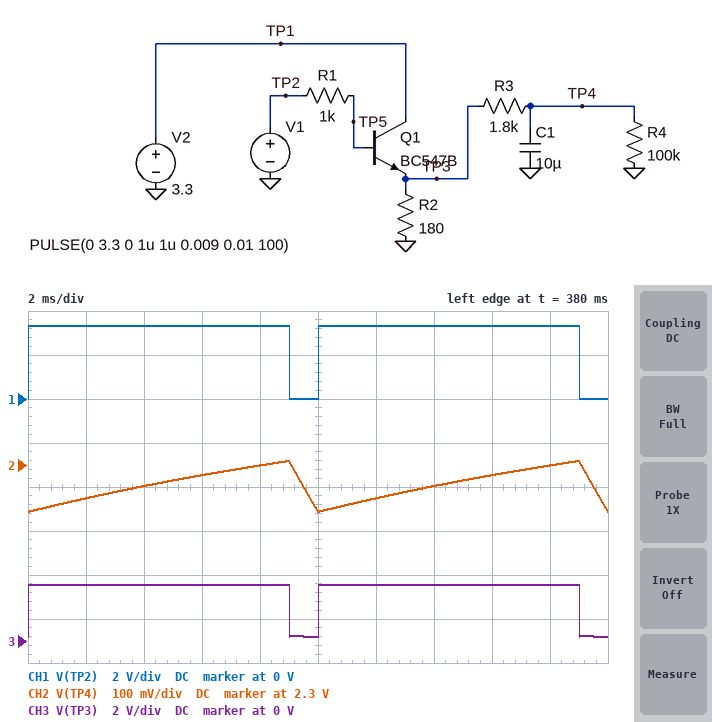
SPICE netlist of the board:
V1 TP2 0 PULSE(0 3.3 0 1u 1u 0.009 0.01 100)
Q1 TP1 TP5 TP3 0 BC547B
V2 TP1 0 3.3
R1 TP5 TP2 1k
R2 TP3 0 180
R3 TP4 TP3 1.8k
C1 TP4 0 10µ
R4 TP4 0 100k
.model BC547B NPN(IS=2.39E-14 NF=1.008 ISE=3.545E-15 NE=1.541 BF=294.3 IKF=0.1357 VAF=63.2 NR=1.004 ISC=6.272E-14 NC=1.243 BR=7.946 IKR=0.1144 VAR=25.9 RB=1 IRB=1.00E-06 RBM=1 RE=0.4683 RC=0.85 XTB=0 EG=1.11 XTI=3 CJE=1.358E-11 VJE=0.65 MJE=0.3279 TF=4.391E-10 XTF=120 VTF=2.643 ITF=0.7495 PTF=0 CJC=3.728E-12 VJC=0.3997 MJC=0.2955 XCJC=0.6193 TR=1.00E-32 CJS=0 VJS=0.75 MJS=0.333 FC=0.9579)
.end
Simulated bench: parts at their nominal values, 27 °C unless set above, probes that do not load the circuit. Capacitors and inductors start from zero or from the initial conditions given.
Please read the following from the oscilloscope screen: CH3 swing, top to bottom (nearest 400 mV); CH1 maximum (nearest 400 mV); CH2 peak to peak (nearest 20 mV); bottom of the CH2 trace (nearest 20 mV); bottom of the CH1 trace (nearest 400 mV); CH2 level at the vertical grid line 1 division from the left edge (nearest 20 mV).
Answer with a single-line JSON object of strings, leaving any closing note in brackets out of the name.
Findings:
{"CH3 swing, top to bottom": "2.4 V", "CH1 maximum": "3.2 V", "CH2 peak to peak": "120 mV", "bottom of the CH2 trace": "2.20 V", "bottom of the CH1 trace": "0 V", "CH2 level at the vertical grid line 1 division from the left edge": "2.22 V"}
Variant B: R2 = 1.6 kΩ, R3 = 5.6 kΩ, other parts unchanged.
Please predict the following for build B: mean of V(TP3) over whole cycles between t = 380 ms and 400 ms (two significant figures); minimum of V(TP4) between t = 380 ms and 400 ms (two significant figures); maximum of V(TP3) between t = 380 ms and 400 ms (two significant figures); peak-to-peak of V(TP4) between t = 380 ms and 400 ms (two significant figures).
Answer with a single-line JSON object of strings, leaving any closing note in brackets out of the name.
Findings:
{"mean of V(TP3) over whole cycles between t = 380 ms and 400 ms": "2.4 V", "minimum of V(TP4) between t = 380 ms and 400 ms": "2.3 V", "maximum of V(TP3) between t = 380 ms and 400 ms": "2.6 V", "peak-to-peak of V(TP4) between t = 380 ms and 400 ms": "35 mV"}
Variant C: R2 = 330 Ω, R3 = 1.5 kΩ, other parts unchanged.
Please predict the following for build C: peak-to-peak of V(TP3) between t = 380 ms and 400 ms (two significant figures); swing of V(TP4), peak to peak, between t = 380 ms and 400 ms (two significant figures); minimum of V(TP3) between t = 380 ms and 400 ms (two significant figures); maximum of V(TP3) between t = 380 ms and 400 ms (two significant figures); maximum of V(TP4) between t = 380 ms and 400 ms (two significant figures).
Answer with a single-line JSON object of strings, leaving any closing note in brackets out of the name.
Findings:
{"peak-to-peak of V(TP3) between t = 380 ms and 400 ms": "2.2 V", "swing of V(TP4), peak to peak, between t = 380 ms and 400 ms": "130 mV", "minimum of V(TP3) between t = 380 ms and 400 ms": "410 mV", "maximum of V(TP3) between t = 380 ms and 400 ms": "2.6 V", "maximum of V(TP4) between t = 380 ms and 400 ms": "2.4 V"}
